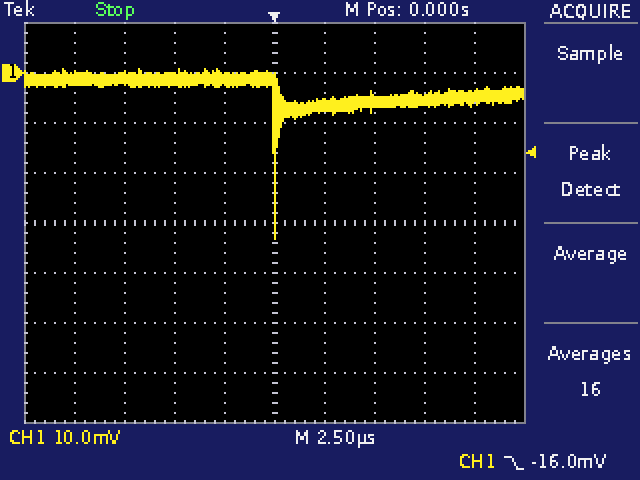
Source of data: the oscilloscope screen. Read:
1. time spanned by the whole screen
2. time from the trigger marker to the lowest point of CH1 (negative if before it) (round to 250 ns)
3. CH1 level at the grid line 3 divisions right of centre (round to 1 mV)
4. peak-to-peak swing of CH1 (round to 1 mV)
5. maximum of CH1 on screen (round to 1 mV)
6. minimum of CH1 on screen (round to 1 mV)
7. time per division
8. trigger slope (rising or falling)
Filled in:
25 µs
0.00 µs
-5 mV
34 mV
1 mV
-33 mV
2.5 µs
falling
